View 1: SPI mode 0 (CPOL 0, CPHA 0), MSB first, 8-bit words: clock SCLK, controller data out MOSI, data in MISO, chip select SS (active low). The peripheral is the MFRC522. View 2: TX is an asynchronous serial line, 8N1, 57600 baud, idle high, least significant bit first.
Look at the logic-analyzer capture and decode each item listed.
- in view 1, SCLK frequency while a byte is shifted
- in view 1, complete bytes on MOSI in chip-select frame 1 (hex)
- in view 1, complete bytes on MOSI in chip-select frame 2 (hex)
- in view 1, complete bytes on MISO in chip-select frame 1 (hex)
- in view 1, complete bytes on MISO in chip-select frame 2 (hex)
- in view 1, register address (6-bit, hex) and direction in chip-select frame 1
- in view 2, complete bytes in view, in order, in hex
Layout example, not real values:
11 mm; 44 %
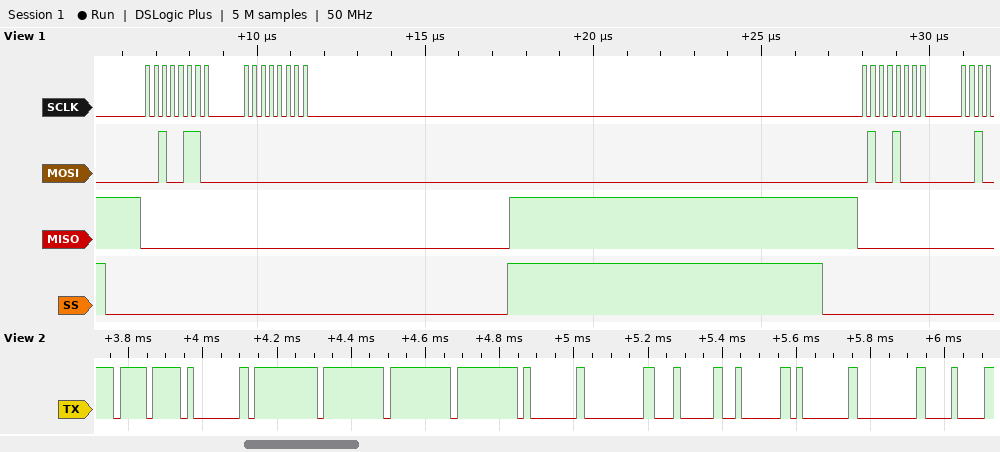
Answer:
4 MHz; 0x26 0x00; 0x48; 0x00 0x00; 0x00; 0x13 write; 0xEF 0x01 0xFF 0xFF 0xFF 0xFF 0x01 0x00 0x04 0x02 0x01 0x00 0x08
